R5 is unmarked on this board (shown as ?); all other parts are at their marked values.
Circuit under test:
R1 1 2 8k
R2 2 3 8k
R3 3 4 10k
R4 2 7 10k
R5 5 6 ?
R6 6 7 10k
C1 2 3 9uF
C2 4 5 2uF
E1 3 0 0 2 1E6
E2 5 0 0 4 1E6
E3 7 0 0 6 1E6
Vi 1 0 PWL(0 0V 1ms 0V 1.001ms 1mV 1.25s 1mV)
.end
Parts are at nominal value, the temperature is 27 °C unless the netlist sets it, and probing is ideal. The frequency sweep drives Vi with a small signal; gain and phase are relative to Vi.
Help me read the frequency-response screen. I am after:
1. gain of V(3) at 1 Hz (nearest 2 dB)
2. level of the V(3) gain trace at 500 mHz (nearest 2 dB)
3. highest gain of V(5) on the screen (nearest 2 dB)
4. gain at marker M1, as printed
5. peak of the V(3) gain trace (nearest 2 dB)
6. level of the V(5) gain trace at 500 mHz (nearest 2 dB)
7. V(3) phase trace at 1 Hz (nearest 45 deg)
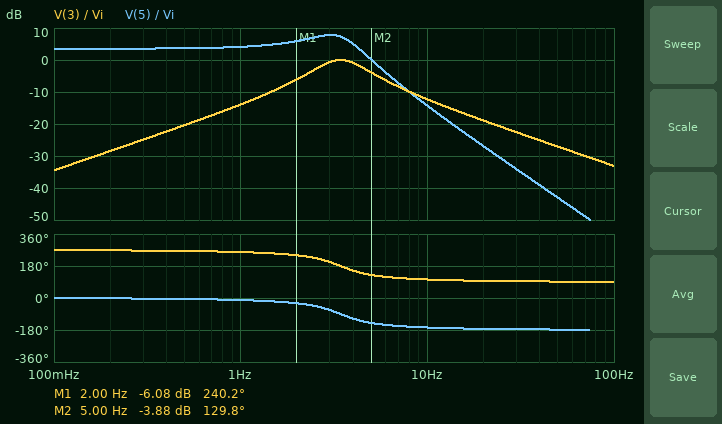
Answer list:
-14 dB
-20 dB
8 dB
-6.08 dB
0 dB
4 dB
270 deg
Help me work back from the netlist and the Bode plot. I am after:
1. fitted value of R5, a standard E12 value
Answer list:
12 kΩ
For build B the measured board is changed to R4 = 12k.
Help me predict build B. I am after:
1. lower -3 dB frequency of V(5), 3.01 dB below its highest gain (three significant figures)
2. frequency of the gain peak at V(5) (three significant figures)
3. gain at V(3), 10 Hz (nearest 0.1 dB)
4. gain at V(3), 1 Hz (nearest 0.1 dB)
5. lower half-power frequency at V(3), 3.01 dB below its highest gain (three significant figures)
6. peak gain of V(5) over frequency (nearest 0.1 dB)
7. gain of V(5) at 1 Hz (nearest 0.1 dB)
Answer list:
930 mHz
2.71 Hz
-12.5 dB
-12.2 dB
2.21 Hz
8.7 dB
5.8 dB
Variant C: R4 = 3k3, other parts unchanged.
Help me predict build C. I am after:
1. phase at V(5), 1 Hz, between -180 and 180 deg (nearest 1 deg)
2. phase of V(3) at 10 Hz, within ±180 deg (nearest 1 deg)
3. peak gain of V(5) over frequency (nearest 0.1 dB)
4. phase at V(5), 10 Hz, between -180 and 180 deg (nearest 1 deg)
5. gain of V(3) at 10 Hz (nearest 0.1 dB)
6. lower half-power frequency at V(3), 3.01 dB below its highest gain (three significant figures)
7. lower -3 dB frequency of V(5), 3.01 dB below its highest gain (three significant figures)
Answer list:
-4 deg
109 deg
2.7 dB
-161 deg
-9.8 dB
4.96 Hz
4.49 Hz
